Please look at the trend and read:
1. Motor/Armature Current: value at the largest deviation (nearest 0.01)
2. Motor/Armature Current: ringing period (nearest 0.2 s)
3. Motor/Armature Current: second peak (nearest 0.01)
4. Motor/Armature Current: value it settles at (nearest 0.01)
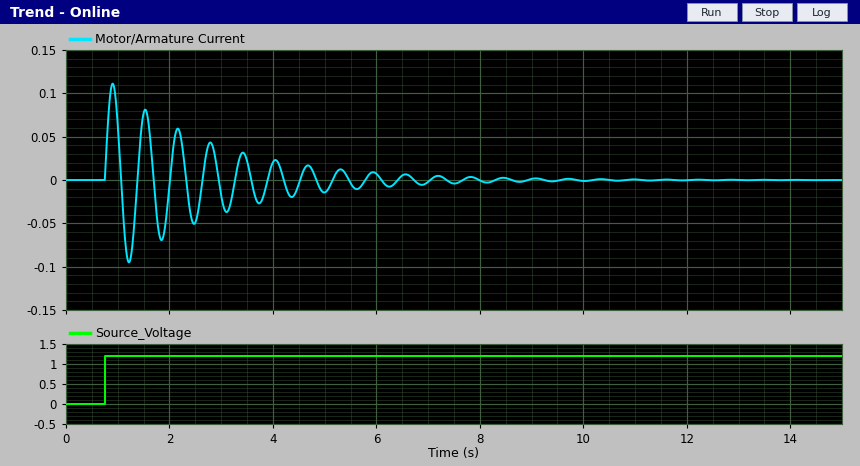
0.11
0.6 s
0.08
0.00
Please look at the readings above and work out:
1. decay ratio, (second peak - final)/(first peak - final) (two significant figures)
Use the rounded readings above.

0.73
